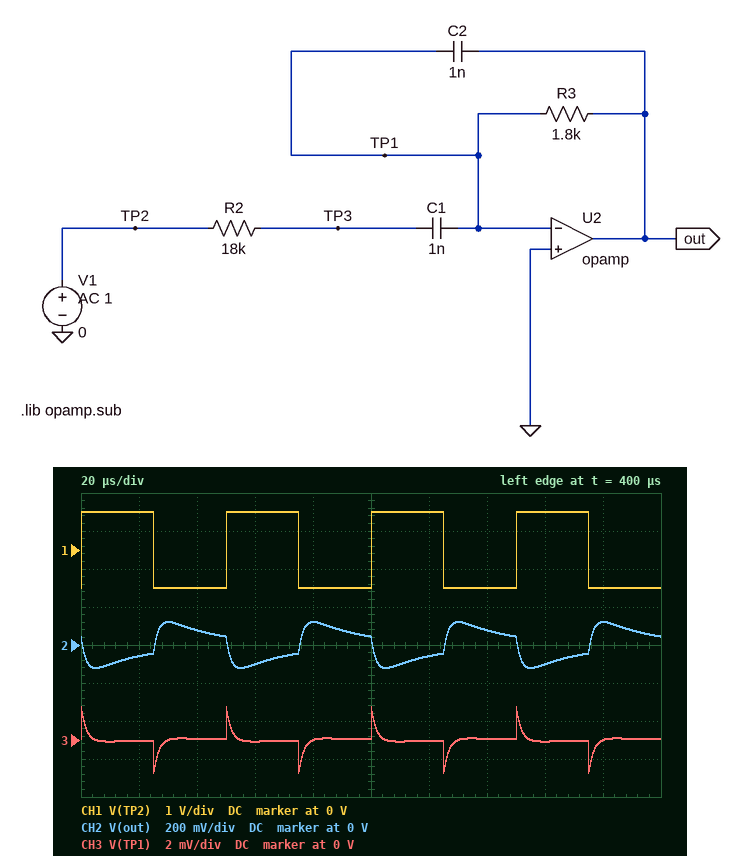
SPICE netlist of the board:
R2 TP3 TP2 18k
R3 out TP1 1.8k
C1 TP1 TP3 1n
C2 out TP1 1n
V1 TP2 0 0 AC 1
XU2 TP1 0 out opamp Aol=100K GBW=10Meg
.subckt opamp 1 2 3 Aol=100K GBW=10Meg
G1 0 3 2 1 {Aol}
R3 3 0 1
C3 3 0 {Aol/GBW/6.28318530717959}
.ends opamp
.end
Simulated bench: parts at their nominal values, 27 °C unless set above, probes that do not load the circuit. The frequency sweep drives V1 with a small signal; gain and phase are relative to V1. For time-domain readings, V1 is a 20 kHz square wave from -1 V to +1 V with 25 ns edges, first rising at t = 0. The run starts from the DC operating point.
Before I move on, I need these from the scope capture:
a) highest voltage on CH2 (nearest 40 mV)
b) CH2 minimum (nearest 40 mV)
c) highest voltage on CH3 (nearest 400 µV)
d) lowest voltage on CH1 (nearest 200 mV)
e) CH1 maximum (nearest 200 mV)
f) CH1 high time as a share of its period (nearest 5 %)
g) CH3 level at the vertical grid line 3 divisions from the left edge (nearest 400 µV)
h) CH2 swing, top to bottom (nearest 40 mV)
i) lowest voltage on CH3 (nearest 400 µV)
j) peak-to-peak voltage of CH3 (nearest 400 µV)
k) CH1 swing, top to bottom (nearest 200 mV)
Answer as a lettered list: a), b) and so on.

a) 120 mV
b) -120 mV
c) 1.6 mV
d) -1.0 V
e) 1.0 V
f) 50 %
g) 0 V
h) 240 mV
i) -1.6 mV
j) 3.6 mV
k) 2.0 V
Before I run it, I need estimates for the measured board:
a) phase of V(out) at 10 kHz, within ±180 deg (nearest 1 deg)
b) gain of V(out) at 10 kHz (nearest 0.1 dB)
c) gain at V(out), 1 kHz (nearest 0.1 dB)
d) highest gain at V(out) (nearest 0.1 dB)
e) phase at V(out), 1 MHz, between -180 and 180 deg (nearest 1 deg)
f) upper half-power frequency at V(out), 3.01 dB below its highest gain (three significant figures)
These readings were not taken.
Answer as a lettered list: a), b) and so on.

a) -145 deg
b) -22.6 dB
c) -39.0 dB
d) -20.8 dB
e) 90 deg
f) 105 kHz
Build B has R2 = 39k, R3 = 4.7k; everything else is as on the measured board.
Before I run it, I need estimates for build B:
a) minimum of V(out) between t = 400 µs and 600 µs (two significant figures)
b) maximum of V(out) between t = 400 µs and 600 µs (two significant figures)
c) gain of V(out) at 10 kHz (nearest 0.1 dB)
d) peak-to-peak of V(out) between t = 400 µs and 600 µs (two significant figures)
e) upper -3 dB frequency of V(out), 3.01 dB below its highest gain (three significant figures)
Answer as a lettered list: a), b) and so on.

a) -110 mV
b) 110 mV
c) -19.4 dB
d) 220 mV
e) 41.3 kHz
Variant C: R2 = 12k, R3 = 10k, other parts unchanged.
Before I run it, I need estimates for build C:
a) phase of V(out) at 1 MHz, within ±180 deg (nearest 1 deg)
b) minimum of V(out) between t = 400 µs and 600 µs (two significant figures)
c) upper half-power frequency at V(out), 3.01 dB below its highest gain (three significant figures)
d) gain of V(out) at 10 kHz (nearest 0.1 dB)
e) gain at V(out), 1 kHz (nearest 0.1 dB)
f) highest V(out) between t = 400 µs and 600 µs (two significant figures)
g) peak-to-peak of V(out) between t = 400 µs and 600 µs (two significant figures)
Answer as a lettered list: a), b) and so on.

a) 86 deg
b) -490 mV
c) 35.1 kHz
d) -7.4 dB
e) -24.1 dB
f) 490 mV
g) 980 mV
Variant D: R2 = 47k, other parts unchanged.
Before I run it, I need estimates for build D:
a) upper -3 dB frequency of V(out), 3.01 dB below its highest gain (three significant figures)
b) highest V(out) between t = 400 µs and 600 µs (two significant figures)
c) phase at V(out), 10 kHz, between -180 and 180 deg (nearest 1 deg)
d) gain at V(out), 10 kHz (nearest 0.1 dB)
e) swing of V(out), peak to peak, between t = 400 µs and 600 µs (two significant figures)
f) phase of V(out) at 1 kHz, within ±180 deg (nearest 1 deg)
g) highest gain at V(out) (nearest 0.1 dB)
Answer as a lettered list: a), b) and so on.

a) 94.9 kHz
b) 42 mV
c) -168 deg
d) -28.9 dB
e) 83 mV
f) -107 deg
g) -28.7 dB
